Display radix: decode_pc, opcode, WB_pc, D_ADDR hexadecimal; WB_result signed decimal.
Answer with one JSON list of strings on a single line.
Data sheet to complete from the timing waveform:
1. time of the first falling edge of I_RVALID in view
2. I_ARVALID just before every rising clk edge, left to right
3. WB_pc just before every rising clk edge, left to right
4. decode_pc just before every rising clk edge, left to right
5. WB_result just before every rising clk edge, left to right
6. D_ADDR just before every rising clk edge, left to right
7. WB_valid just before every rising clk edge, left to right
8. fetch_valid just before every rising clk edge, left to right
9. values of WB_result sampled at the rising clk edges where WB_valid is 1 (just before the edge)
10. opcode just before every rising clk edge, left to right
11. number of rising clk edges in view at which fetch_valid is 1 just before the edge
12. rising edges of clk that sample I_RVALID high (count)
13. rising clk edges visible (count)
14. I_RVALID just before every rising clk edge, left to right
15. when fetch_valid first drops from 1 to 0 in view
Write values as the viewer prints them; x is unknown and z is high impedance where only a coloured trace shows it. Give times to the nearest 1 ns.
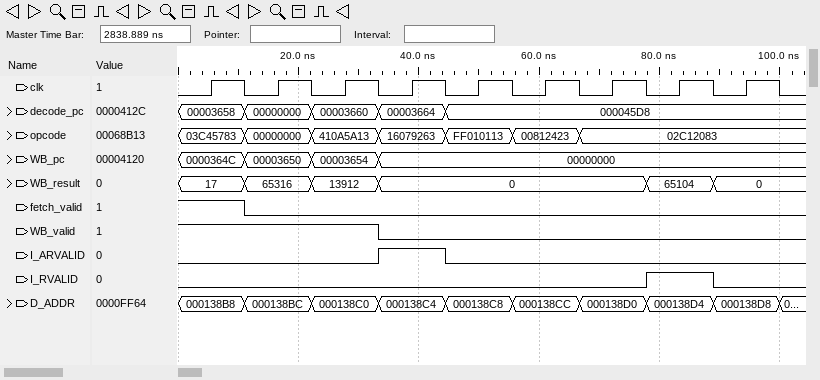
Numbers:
["89 ns", "0 0 0 1 0 0 0 0 0", "0000364C, 00003650, 00003654, 00000000, 00000000, 00000000, 00000000, 00000000, 00000000", "00003658, 00000000, 00003660, 00003664, 000045D8, 000045D8, 000045D8, 000045D8, 000045D8", "17, 65316, 13912, 0, 0, 0, 0, 65104, 0", "000138B8, 000138BC, 000138C0, 000138C4, 000138C8, 000138CC, 000138D0, 000138D4, 000138D8", "1 1 1 0 0 0 0 0 0", "1 0 0 0 0 0 0 0 0", "17, 65316, 13912", "03C45783, 00000000, 410A5A13, 16079263, FF010113, 00812423, 02C12083, 02C12083, 02C12083", "1", "1", "9", "0 0 0 0 0 0 0 1 0", "11 ns"]
